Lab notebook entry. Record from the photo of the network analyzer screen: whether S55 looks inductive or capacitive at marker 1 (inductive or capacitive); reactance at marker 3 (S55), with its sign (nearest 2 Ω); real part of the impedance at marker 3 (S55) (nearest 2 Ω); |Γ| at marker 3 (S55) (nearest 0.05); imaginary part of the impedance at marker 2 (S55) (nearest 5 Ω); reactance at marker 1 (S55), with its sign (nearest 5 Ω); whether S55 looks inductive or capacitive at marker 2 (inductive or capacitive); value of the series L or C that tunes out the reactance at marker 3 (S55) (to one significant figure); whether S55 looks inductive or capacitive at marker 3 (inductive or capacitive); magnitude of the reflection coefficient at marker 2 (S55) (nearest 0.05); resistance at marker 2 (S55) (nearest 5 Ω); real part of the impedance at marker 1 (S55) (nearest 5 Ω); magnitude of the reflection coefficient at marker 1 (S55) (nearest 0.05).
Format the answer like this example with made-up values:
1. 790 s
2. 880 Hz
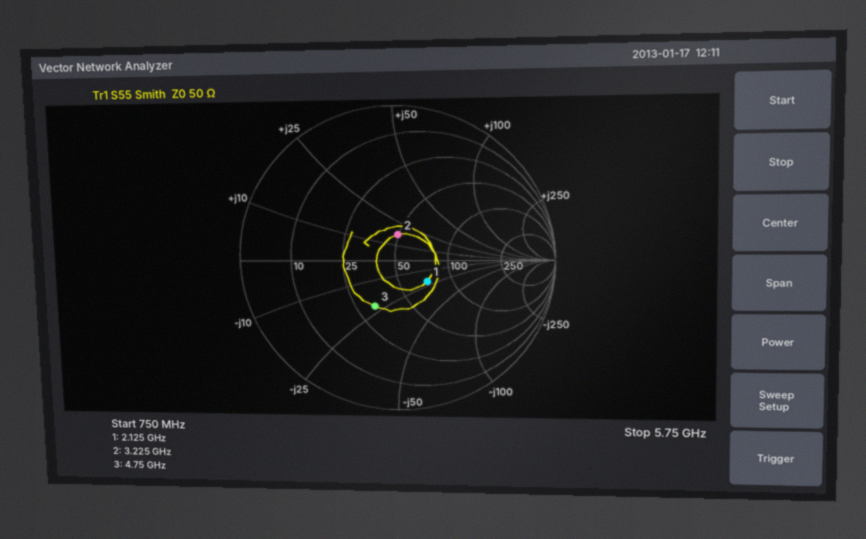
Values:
1. capacitive
2. -22 Ω
3. 32 Ω
4. 0.35
5. +15 Ω
6. -20 Ω
7. inductive
8. 700 pH
9. capacitive
10. 0.15
11. 50 Ω
12. 70 Ω
13. 0.25
